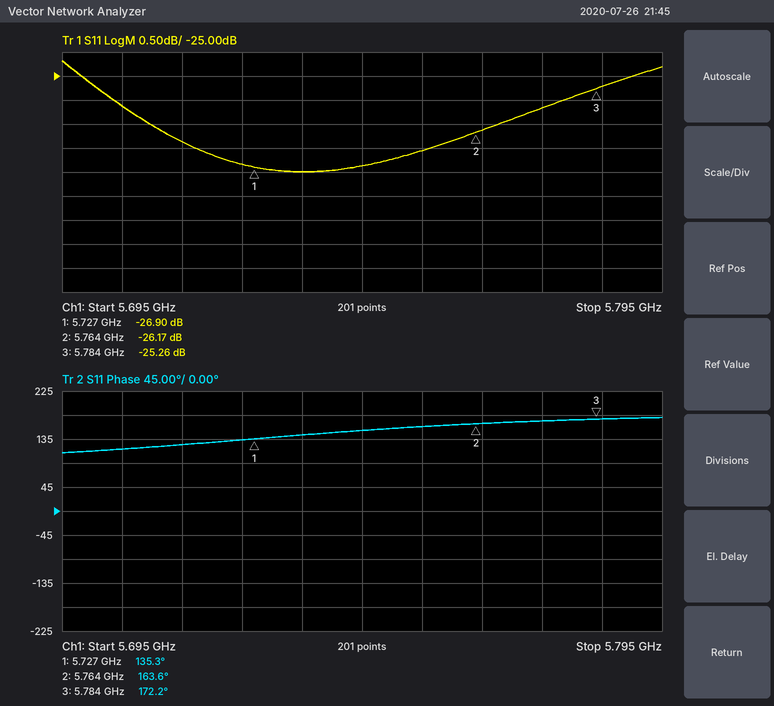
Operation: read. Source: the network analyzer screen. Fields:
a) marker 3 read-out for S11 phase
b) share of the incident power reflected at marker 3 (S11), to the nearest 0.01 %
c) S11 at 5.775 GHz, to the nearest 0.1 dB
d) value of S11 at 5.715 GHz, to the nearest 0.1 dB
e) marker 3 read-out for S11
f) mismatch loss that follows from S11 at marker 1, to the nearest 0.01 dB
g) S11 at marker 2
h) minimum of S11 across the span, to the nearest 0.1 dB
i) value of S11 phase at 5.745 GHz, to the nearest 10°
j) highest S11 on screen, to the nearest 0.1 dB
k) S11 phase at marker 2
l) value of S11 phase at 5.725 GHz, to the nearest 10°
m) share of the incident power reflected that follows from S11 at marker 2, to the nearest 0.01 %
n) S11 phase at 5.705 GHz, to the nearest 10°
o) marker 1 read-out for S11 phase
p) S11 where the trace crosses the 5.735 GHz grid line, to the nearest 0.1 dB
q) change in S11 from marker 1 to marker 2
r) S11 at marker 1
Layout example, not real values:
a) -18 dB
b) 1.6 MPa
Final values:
a) 172.2°
b) 0.30 %
c) -25.7 dB
d) -26.4 dB
e) -25.26 dB
f) 0.01 dB
g) -26.17 dB
h) -27.0 dB
i) 150°
j) -24.7 dB
k) 163.6°
l) 130°
m) 0.24 %
n) 120°
o) 135.3°
p) -27.0 dB
q) 0.73 dB
r) -26.90 dB
